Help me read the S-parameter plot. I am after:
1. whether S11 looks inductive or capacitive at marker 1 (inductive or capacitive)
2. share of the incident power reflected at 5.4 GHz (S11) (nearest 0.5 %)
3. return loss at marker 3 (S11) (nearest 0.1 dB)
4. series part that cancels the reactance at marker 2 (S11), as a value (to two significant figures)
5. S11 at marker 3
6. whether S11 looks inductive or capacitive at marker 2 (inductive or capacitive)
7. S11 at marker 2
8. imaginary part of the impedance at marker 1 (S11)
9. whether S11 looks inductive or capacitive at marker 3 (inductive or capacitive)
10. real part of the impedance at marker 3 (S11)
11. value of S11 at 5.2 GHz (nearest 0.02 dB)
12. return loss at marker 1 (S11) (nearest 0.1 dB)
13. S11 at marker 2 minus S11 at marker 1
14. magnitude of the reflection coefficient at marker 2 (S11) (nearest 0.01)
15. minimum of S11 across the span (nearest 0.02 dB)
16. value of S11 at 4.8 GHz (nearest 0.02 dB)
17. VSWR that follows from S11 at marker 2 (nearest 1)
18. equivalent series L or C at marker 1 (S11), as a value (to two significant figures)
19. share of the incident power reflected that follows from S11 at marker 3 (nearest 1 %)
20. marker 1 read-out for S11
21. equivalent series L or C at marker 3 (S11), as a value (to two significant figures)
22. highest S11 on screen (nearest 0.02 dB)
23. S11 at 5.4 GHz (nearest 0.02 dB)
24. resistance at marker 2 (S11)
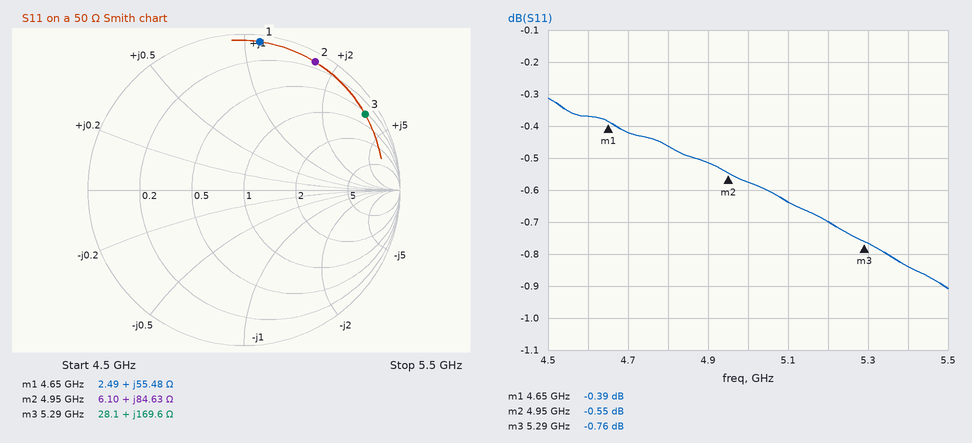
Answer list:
inductive
82.5 %
0.8 dB
380 fF
-0.76 dB
inductive
-0.55 dB
+55.48 Ω
inductive
28.1 Ω
-0.70 dB
0.4 dB
-0.16 dB
0.94
-0.90 dB
-0.46 dB
32
1.9 nH
84 %
-0.39 dB
5.1 nH
-0.32 dB
-0.84 dB
6.10 Ω
